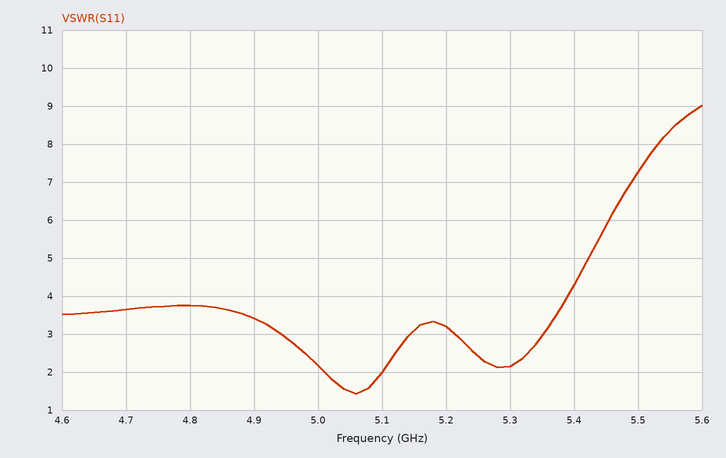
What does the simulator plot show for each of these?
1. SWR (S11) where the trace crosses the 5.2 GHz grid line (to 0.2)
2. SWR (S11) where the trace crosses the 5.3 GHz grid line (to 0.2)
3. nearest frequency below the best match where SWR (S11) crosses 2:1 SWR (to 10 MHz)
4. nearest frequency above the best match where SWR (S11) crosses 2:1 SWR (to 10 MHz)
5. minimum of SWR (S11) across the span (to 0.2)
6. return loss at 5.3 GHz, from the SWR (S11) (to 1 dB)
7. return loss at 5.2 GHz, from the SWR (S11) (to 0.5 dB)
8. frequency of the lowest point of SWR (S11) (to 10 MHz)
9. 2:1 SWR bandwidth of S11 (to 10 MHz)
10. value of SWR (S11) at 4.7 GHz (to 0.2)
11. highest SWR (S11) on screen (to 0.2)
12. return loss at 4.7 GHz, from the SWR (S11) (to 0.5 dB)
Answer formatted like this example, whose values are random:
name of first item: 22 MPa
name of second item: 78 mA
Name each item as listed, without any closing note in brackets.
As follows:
SWR (S11) where the trace crosses the 5.2 GHz grid line: 3.2
SWR (S11) where the trace crosses the 5.3 GHz grid line: 2.2
nearest frequency below the best match where SWR (S11) crosses 2:1 SWR: 5.01 GHz
nearest frequency above the best match where SWR (S11) crosses 2:1 SWR: 5.10 GHz
minimum of SWR (S11) across the span: 1.4
return loss at 5.3 GHz, from the SWR (S11): 9 dB
return loss at 5.2 GHz, from the SWR (S11): 5.5 dB
frequency of the lowest point of SWR (S11): 5.06 GHz
2:1 SWR bandwidth of S11: 90 MHz
value of SWR (S11) at 4.7 GHz: 3.6
highest SWR (S11) on screen: 9.0
return loss at 4.7 GHz, from the SWR (S11): 5.0 dB
